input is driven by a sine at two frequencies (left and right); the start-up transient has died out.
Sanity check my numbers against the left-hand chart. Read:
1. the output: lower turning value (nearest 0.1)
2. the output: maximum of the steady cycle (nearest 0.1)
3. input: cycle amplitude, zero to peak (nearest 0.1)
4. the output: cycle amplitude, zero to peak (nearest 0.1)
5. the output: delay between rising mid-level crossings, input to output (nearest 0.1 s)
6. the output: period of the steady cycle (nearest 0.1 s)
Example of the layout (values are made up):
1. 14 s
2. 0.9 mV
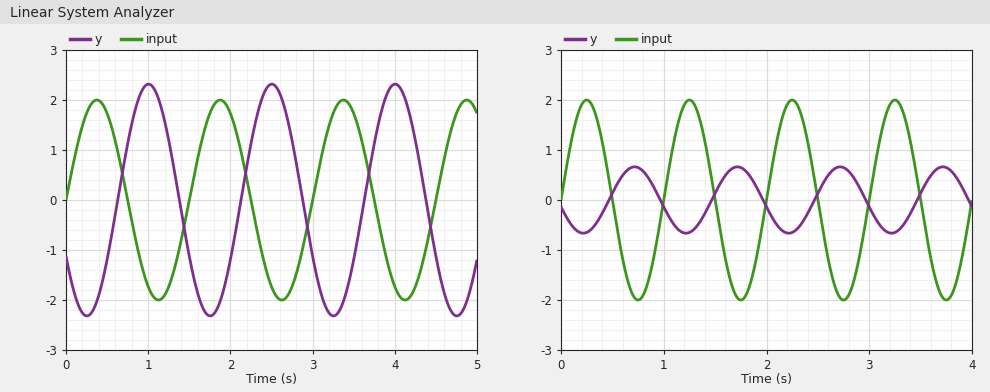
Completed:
1. -2.3
2. 2.3
3. 2.0
4. 2.3
5. 0.6 s
6. 1.5 s
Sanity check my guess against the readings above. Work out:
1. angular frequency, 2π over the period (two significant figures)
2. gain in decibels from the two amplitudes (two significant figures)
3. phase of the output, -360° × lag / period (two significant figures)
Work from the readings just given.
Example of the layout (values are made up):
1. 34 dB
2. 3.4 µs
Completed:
1. 4.2 rad/s
2. 1.2 dB
3. -140°
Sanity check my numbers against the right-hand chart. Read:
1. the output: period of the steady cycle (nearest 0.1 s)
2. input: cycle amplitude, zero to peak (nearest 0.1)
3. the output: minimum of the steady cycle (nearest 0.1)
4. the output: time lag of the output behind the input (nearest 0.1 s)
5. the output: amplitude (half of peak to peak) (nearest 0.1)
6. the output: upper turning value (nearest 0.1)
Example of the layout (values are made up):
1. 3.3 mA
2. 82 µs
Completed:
1. 1.0 s
2. 2.0
3. -0.7
4. 0.5 s
5. 0.7
6. 0.7
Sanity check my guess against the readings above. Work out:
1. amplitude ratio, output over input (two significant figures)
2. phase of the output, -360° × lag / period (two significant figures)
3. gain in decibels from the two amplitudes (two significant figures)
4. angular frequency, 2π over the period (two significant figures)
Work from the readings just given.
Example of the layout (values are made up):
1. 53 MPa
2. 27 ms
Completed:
1. 0.35
2. -180°
3. -9.1 dB
4. 6.3 rad/s
